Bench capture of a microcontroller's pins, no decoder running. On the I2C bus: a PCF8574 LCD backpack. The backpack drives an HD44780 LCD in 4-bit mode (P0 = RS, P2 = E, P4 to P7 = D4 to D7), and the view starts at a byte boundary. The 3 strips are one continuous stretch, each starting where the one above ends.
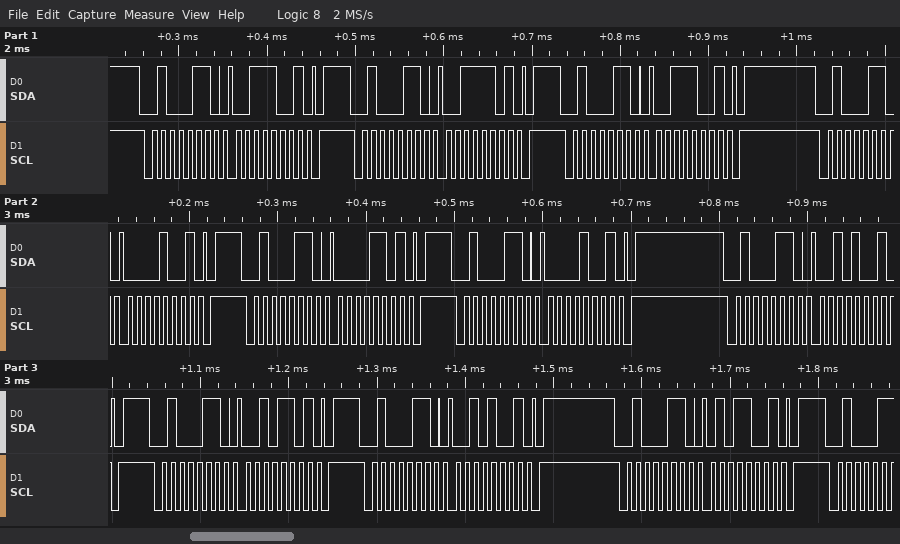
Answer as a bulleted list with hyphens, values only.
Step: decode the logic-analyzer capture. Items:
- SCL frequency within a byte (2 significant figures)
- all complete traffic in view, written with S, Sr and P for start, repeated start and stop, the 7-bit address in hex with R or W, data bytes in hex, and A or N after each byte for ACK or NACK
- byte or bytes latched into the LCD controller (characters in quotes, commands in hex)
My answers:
- 100 kHz
- S 23W A 39 A P S 23W A 3D A P S 23W A 39 A P S 23W A 09 A P S 23W A 0D A P S 23W A 09 A P S 23W A 29 A P S 23W A 2D A P S 23W A 29 A P S 23W A 59 A P
- '0'
